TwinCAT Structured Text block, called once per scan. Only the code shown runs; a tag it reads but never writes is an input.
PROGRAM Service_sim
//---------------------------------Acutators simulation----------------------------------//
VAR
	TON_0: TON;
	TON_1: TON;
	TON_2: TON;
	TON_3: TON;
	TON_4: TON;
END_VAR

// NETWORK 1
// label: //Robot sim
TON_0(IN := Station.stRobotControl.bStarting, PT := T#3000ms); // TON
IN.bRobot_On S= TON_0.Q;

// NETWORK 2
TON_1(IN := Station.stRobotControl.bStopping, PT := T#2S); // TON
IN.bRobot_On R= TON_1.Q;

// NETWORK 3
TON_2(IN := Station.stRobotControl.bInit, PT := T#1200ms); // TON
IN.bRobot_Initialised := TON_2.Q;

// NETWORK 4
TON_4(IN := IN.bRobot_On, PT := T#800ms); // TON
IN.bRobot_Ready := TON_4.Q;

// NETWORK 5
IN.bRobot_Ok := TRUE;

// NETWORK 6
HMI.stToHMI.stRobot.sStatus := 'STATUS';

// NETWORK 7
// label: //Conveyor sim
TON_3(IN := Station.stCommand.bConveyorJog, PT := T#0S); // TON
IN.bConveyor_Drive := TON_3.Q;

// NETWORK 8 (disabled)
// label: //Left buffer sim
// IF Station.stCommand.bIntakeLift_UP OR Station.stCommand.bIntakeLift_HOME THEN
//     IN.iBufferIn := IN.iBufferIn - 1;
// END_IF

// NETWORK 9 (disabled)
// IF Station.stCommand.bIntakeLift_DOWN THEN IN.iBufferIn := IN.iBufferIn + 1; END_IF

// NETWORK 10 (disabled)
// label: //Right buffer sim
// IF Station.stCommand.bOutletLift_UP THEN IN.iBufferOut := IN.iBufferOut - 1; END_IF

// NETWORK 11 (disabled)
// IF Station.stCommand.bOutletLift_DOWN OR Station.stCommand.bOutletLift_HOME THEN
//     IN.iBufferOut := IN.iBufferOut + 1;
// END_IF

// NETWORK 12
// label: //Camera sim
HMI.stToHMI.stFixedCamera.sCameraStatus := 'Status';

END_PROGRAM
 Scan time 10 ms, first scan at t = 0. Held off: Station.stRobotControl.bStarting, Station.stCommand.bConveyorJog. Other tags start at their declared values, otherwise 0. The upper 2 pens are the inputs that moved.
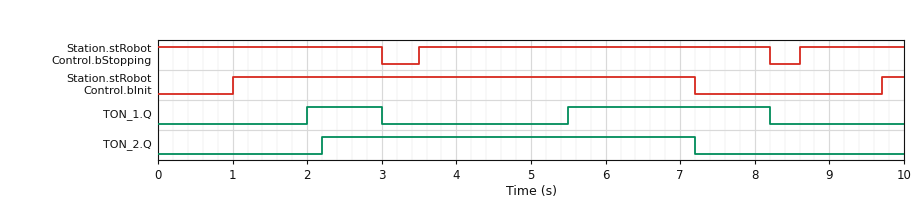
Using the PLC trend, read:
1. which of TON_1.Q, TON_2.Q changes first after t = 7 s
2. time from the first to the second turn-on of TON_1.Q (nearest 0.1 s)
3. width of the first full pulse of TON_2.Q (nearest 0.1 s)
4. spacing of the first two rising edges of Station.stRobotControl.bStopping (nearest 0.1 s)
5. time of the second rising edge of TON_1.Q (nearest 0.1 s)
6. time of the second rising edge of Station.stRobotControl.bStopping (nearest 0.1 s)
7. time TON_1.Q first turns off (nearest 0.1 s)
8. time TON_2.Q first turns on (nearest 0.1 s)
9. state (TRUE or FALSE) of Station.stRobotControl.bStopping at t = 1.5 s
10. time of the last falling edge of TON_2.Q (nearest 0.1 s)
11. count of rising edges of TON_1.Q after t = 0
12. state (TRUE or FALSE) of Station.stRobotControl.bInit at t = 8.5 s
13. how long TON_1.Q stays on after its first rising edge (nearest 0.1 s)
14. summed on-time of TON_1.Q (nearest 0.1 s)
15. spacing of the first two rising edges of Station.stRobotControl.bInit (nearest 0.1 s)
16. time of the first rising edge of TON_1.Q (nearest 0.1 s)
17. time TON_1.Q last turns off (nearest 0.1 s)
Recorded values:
TON_2.Q
3.5 s
5.0 s
5.1 s
5.5 s
8.6 s
3.0 s
2.2 s
TRUE
7.2 s
2
FALSE
1.0 s
3.7 s
8.7 s
2.0 s
8.2 s
